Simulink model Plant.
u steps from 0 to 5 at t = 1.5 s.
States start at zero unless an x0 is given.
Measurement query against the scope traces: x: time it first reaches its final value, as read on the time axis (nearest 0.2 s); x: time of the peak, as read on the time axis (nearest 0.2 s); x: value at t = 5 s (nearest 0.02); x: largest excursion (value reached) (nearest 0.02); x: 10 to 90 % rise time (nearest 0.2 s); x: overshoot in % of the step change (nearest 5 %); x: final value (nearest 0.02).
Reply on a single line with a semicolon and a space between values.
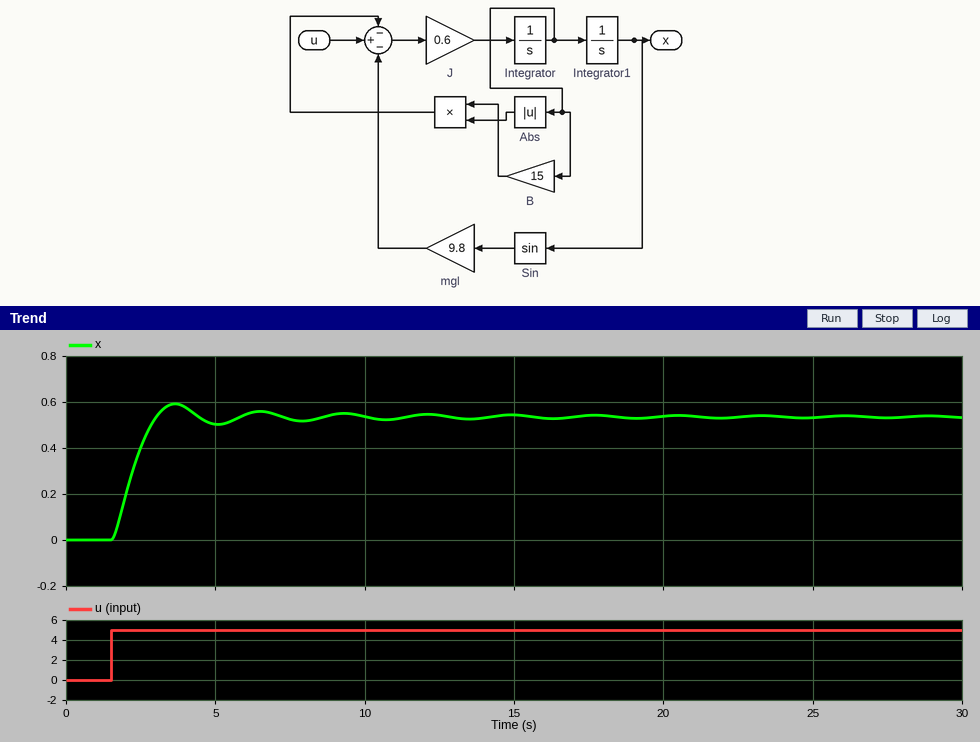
3.0 s; 3.6 s; 0.50; 0.60; 1.0 s; 10 %; 0.54
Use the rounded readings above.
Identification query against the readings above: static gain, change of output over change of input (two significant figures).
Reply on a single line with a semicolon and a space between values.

0.11
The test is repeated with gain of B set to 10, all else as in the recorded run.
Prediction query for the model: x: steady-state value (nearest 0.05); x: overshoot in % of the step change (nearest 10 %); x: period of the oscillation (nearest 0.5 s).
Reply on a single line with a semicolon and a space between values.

0.55; 20 %; 3.0 s
